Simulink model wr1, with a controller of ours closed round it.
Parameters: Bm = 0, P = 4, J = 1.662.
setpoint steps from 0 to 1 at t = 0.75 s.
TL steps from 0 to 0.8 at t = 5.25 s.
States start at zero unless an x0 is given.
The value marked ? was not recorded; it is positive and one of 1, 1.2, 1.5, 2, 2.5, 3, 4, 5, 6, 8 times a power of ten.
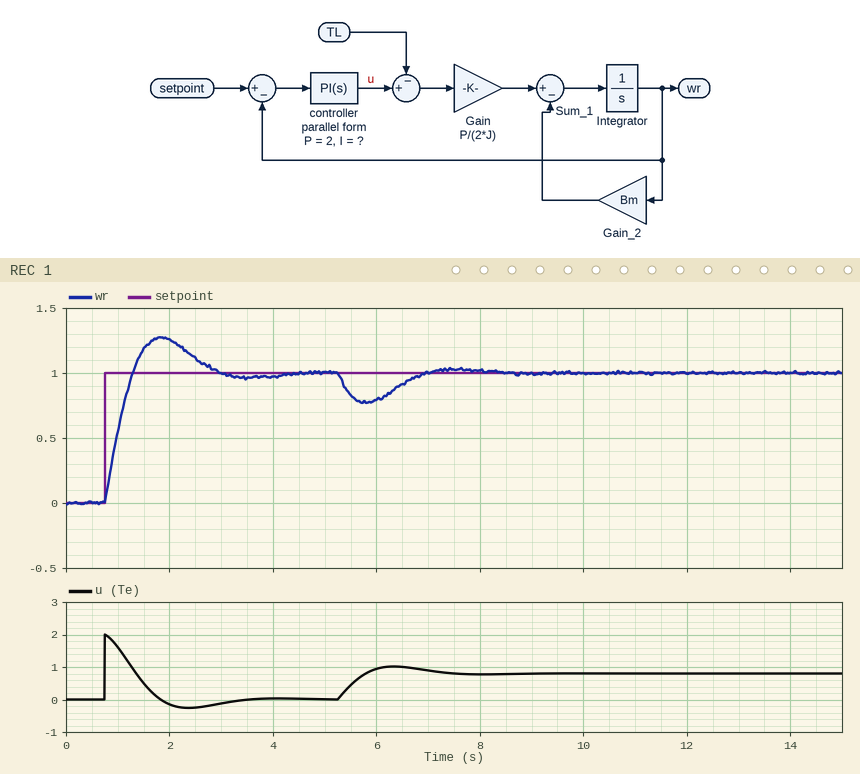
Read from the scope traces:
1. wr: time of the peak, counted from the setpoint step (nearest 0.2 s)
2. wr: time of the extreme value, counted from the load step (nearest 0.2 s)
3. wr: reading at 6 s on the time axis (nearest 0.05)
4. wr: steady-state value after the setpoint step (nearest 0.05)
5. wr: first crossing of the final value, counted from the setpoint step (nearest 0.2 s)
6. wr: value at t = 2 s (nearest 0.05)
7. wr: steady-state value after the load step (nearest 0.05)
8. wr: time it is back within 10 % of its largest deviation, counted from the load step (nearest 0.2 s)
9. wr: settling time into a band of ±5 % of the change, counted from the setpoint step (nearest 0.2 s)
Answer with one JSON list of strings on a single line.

["1.0 s", "0.6 s", "0.80", "1.00", "0.6 s", "1.25", "1.00", "2.6 s", "2.0 s"]
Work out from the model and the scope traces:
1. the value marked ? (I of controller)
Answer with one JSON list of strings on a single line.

["4"]
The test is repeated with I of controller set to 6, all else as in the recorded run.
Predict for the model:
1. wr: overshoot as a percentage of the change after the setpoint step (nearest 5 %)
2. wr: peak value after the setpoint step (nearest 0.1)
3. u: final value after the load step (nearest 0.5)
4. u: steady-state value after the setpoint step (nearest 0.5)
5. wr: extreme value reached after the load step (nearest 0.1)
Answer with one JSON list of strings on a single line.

["35 %", "1.3", "1.0", "0.0", "0.8"]
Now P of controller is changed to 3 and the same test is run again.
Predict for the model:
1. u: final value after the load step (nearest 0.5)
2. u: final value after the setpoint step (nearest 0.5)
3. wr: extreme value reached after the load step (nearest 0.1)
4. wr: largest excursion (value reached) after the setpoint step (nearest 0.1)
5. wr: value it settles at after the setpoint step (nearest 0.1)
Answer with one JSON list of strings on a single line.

["1.0", "0.0", "0.8", "1.2", "1.0"]
